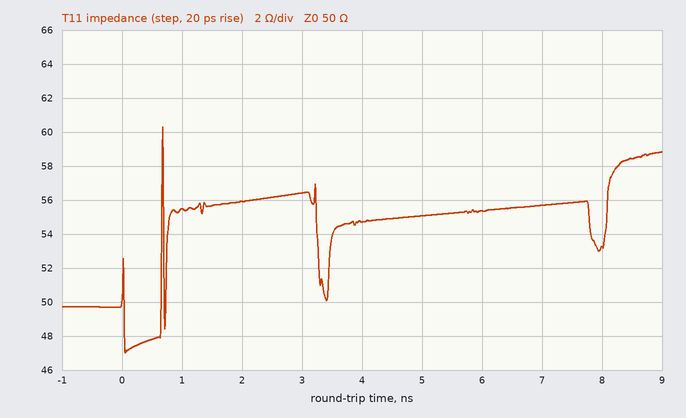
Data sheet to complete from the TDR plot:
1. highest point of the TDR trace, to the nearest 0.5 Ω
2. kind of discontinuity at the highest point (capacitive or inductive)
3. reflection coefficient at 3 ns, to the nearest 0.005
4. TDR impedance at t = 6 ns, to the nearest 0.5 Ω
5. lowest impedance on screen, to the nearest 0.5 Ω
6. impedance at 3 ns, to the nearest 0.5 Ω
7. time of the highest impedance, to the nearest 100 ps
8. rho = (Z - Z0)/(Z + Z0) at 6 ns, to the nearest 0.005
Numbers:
60.5 Ω
inductive
+0.060
55.5 Ω
47.0 Ω
56.5 Ω
700 ps
+0.050
